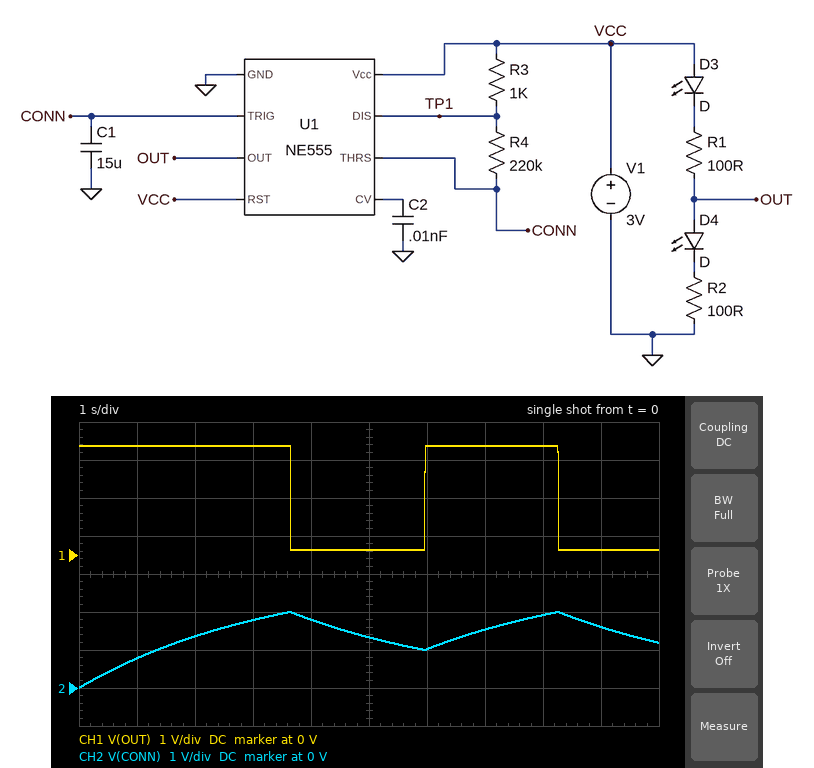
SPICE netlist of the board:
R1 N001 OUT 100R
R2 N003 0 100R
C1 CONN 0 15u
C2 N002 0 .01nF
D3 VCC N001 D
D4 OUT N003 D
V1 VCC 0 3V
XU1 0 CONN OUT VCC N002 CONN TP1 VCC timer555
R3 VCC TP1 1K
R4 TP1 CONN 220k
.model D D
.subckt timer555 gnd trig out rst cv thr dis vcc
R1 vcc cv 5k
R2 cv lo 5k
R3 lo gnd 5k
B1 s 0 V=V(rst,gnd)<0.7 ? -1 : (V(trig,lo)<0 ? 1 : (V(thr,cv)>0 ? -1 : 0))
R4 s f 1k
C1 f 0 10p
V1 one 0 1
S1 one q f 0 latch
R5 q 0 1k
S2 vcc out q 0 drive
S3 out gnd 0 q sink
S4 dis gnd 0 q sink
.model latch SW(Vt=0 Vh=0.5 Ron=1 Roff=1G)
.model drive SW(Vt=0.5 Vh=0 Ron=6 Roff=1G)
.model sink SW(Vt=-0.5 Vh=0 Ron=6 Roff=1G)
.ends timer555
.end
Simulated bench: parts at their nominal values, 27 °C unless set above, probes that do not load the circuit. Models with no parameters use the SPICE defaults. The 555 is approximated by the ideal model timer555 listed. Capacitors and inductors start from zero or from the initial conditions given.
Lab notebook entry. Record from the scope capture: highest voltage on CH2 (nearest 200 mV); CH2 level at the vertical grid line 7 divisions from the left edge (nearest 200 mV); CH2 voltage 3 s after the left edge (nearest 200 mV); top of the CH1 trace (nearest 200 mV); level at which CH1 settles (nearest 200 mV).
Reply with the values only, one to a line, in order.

2.0 V
1.6 V
1.8 V
2.8 V
200 mV
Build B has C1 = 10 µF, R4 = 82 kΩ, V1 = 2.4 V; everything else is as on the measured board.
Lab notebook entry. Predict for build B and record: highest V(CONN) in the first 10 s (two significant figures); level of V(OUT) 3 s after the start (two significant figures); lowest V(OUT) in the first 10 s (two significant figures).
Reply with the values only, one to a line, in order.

1.6 V
2.3 V
95 mV
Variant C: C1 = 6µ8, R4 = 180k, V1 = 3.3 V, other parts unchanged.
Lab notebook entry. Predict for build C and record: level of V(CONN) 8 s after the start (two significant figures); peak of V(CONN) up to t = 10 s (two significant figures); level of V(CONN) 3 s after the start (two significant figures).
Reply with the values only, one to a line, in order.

2.0 V
2.2 V
2.1 V
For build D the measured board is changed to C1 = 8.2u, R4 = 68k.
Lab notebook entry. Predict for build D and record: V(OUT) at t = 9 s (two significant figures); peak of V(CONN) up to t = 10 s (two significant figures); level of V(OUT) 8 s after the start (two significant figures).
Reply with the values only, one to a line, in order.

2.9 V
2.0 V
130 mV
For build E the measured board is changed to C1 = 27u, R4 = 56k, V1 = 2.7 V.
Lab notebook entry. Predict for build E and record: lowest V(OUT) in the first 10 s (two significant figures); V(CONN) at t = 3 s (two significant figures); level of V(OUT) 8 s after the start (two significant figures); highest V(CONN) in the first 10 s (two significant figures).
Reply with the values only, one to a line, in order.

110 mV
1.2 V
2.6 V
1.8 V
